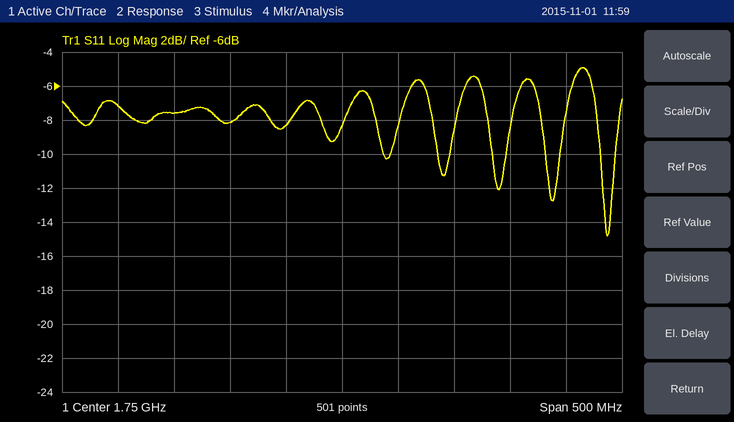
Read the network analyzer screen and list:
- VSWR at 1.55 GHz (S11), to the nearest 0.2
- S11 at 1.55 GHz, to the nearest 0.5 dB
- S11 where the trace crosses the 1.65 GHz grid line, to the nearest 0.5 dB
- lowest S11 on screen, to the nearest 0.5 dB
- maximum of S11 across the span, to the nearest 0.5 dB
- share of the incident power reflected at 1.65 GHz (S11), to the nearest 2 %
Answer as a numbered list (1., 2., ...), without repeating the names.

1. 2.6
2. -7.0 dB
3. -8.0 dB
4. -15.0 dB
5. -5.0 dB
6. 16 %
